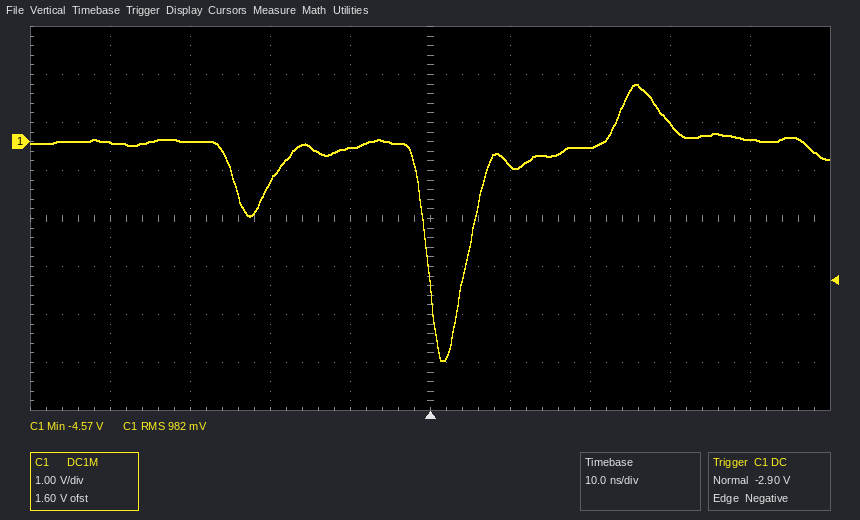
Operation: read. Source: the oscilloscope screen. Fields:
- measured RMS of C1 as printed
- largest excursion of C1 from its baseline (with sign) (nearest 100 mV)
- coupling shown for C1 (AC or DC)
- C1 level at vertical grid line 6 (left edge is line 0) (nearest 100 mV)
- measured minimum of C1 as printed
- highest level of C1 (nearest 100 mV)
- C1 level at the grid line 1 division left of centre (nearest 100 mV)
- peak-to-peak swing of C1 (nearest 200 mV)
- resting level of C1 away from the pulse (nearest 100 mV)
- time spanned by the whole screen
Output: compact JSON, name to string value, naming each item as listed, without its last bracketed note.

{"measured RMS of C1 as printed": "982 mV", "largest excursion of C1 from its baseline (with sign)": "-4.6 V", "coupling shown for C1": "DC", "C1 level at vertical grid line 6 (left edge is line 0)": "-500 mV", "measured minimum of C1 as printed": "-4.57 V", "highest level of C1": "1.2 V", "C1 level at the grid line 1 division left of centre": "-100 mV", "peak-to-peak swing of C1": "5.8 V", "resting level of C1 away from the pulse": "0.0 V", "time spanned by the whole screen": "100 ns"}
